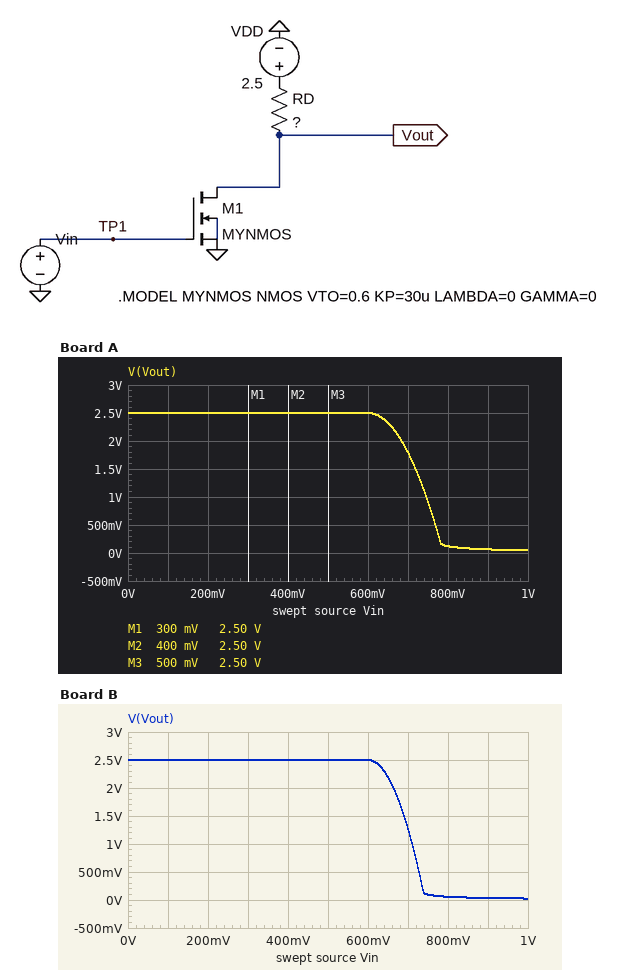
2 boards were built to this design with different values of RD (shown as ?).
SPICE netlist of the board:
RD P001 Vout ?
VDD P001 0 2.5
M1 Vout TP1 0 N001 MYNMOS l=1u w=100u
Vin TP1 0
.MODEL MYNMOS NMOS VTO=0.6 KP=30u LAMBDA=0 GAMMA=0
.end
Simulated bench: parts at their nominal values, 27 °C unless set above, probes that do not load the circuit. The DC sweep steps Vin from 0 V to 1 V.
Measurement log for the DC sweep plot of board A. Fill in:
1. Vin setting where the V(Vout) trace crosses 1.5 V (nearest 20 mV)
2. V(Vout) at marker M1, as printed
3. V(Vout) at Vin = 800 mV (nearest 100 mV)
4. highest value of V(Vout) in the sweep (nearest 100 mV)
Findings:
720 mV
2.50 V
100 mV
2.5 V
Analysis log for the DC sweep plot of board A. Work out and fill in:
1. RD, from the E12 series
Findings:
47 kΩ
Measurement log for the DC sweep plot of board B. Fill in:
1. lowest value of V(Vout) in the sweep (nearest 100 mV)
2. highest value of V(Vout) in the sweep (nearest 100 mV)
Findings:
0 V
2.5 V
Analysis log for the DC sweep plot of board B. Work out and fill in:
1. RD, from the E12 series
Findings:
82 kΩ
